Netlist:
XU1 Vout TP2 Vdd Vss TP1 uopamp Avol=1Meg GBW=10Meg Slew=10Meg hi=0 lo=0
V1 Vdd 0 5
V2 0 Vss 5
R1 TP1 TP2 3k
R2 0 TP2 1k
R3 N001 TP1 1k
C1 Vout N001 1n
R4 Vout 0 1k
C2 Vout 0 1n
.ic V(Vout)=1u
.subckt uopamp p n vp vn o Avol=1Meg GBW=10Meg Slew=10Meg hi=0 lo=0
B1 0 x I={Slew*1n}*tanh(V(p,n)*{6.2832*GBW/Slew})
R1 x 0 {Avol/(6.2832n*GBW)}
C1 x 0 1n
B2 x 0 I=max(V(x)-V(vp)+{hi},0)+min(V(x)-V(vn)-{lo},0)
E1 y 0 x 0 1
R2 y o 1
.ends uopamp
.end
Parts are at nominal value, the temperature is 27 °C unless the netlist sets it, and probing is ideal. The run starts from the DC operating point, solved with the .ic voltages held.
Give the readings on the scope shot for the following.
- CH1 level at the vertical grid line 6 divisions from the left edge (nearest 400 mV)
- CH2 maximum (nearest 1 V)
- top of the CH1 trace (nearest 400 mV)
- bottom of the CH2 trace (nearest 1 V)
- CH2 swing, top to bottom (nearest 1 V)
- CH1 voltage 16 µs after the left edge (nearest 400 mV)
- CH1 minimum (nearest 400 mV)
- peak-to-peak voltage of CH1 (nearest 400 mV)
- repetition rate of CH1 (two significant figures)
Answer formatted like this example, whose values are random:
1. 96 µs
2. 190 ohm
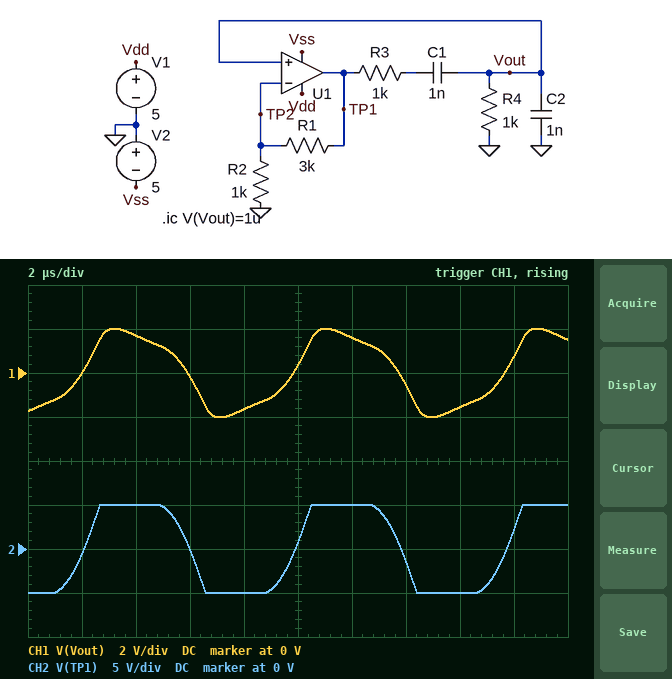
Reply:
1. 1.6 V
2. 5 V
3. 2.0 V
4. -5 V
5. 10 V
6. -1.6 V
7. -2.0 V
8. 4.0 V
9. 130 kHz
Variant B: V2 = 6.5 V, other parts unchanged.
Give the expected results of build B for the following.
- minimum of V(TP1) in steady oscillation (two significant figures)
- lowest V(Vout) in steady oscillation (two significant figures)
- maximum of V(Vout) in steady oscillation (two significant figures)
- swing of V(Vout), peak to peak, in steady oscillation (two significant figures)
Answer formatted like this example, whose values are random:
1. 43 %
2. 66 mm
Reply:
1. -6.5 V
2. -2.4 V
3. 2.2 V
4. 4.6 V
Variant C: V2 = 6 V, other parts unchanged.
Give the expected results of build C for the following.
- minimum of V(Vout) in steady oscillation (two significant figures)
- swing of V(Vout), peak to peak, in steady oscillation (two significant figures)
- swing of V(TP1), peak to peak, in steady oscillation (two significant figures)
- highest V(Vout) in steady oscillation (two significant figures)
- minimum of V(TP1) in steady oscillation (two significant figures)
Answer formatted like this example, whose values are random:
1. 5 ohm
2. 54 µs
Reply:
1. -2.3 V
2. 4.4 V
3. 11 V
4. 2.2 V
5. -6.0 V
